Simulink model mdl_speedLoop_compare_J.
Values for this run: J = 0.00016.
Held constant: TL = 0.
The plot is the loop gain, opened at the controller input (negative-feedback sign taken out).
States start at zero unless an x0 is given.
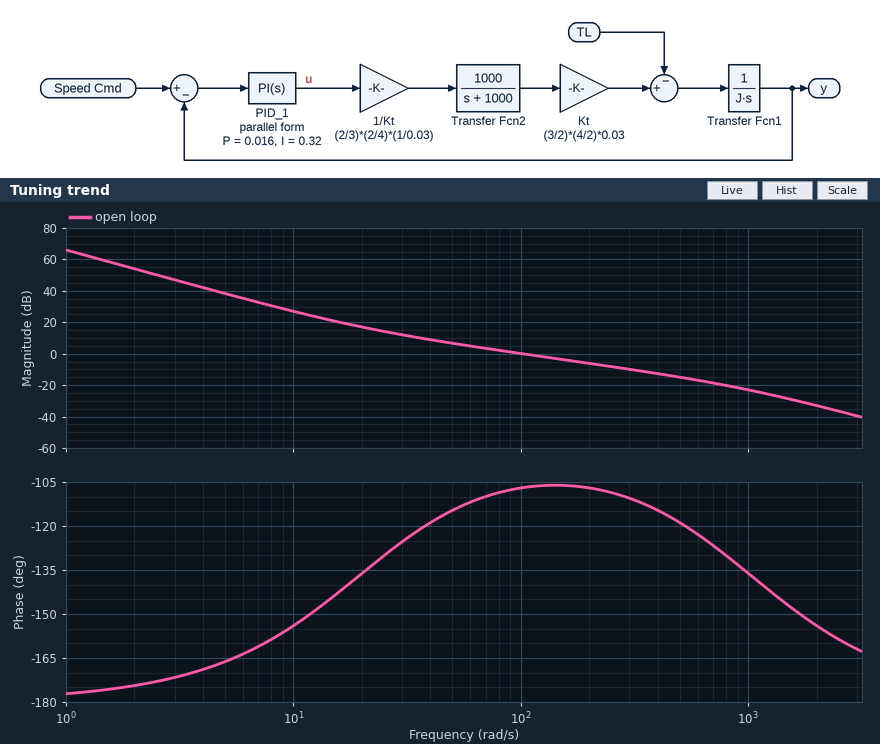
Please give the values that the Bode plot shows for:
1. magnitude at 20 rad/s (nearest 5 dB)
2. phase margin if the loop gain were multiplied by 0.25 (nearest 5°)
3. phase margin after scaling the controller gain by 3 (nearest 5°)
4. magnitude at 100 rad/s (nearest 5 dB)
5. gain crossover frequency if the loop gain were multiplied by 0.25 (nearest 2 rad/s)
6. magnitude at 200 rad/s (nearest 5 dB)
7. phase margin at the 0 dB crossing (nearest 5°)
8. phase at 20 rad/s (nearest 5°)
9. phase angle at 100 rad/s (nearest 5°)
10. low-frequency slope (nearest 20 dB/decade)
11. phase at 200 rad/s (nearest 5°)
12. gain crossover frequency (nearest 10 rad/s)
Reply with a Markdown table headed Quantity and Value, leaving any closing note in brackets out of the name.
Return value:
| Quantity | Value |
|---|---|
| magnitude at 20 rad/s | 15 dB |
| phase margin if the loop gain were multiplied by 0.25 | 55° |
| phase margin after scaling the controller gain by 3 | 70° |
| magnitude at 100 rad/s | 0 dB |
| gain crossover frequency if the loop gain were multiplied by 0.25 | 30 rad/s |
| magnitude at 200 rad/s | -5 dB |
| phase margin at the 0 dB crossing | 75° |
| phase at 20 rad/s | -135° |
| phase angle at 100 rad/s | -105° |
| low-frequency slope | -40 dB/decade |
| phase at 200 rad/s | -105° |
| gain crossover frequency | 100 rad/s |
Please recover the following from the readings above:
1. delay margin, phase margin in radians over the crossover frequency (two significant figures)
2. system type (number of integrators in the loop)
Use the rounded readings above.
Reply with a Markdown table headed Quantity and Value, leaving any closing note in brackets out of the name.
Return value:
| Quantity | Value |
|---|---|
| delay margin, phase margin in radians over the crossover frequency | 0.013 s |
| system type | 2 |
